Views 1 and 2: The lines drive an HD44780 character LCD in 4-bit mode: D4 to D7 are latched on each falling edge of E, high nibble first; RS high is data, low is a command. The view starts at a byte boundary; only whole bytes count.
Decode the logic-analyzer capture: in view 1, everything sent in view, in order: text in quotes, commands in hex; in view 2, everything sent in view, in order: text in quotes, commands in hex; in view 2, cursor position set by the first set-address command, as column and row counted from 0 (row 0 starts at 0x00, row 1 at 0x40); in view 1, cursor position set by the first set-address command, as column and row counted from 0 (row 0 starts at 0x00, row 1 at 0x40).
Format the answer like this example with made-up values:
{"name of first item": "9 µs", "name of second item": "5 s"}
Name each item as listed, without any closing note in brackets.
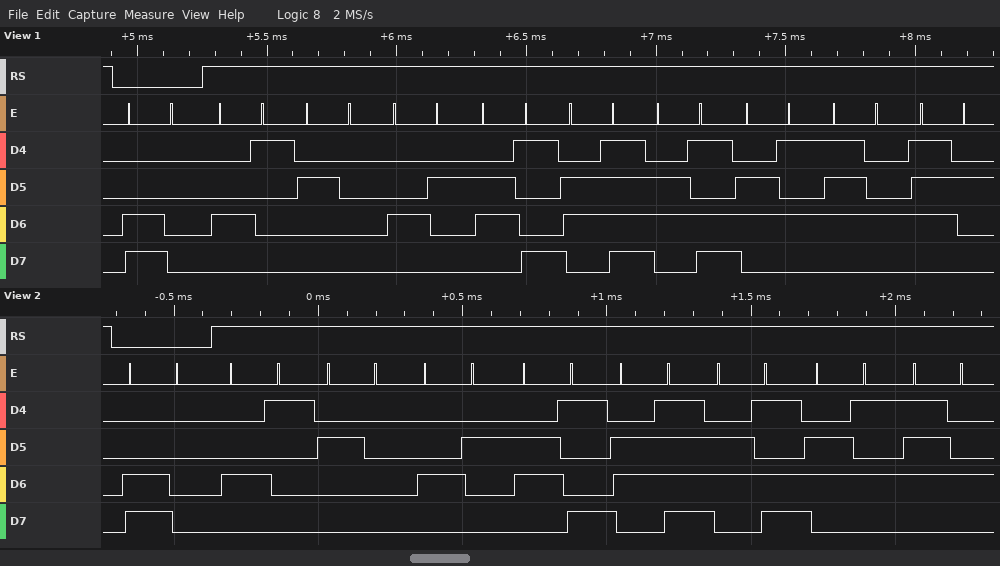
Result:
{"in view 1, everything sent in view, in order: text in quotes, commands in hex": "0xC0 \"A Biometr\"", "in view 2, everything sent in view, in order: text in quotes, commands in hex": "0xC0 \"A Biomet\"", "in view 2, cursor position set by the first set-address command, as column and row counted from 0": "column 0, row 1", "in view 1, cursor position set by the first set-address command, as column and row counted from 0": "column 0, row 1"}
